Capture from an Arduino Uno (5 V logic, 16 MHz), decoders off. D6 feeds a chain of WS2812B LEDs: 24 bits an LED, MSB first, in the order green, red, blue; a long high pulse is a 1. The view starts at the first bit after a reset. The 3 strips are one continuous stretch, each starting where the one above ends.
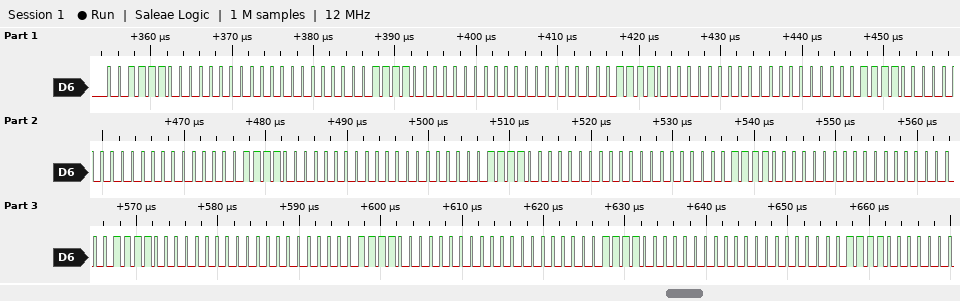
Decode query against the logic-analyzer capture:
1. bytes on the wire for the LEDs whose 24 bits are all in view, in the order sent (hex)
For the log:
3C 00 00 3C 00 00 3C 00 00 3C 00 00 3C 00 00 3C 00 00 3C 00 00 3C 00 00 3C 00 00 3C 00 00
